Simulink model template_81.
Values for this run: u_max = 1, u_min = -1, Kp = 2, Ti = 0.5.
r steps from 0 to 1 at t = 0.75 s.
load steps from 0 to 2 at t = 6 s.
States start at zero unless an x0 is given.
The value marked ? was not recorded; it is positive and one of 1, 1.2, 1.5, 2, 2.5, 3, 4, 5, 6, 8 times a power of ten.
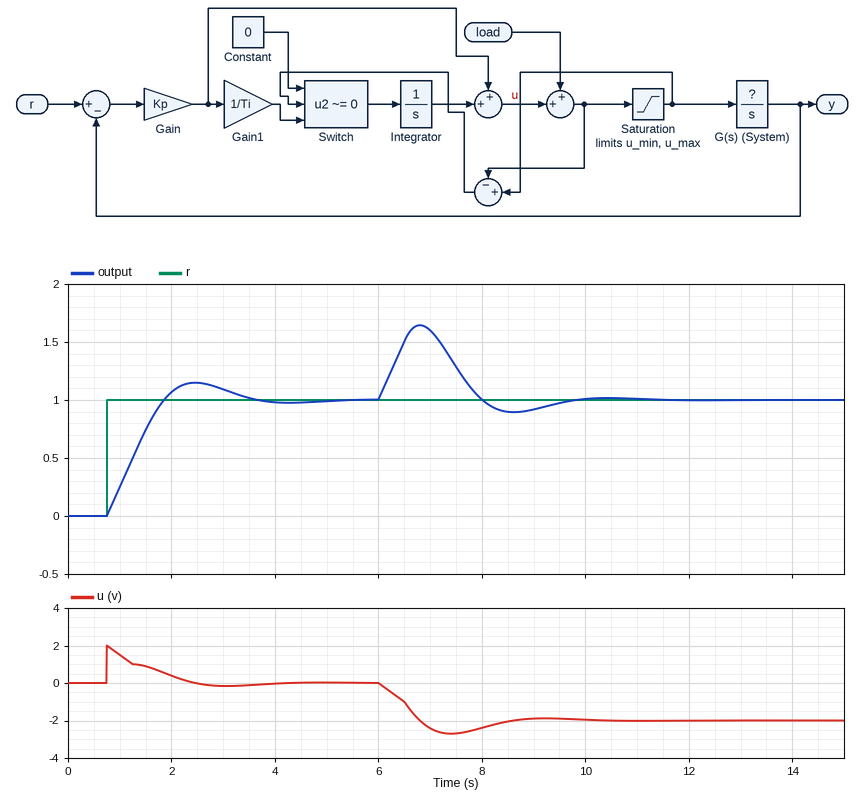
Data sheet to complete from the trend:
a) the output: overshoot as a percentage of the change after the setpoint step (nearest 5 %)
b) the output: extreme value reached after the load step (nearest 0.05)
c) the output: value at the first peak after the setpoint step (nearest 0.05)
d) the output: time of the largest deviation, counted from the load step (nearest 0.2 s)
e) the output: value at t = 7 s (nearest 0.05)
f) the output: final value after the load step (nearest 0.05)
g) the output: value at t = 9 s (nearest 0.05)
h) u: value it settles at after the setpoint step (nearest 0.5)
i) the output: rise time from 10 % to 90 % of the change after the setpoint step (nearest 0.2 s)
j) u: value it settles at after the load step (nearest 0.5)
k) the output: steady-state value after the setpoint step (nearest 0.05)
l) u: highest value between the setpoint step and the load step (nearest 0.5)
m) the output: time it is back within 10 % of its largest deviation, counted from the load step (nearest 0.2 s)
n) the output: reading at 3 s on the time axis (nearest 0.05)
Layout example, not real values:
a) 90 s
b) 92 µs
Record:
a) 15 %
b) 1.65
c) 1.15
d) 0.8 s
e) 1.60
f) 1.00
g) 0.90
h) 0.0
i) 0.8 s
j) -2.0
k) 1.00
l) 2.0
m) 3.2 s
n) 1.10
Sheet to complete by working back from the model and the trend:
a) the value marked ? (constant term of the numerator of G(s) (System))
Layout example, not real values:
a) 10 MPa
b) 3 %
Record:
a) 1
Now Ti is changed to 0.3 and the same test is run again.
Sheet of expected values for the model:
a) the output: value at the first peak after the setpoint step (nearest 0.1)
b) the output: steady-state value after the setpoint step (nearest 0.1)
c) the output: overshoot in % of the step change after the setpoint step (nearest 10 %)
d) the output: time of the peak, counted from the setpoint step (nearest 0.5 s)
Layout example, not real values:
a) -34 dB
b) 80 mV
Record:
a) 1.2
b) 1.0
c) 20 %
d) 1.5 s
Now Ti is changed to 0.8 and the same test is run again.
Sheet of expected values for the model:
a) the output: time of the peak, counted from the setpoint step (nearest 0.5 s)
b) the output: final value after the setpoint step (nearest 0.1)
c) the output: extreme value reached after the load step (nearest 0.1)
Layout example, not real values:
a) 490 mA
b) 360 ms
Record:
a) 2.0 s
b) 1.0
c) 1.7
